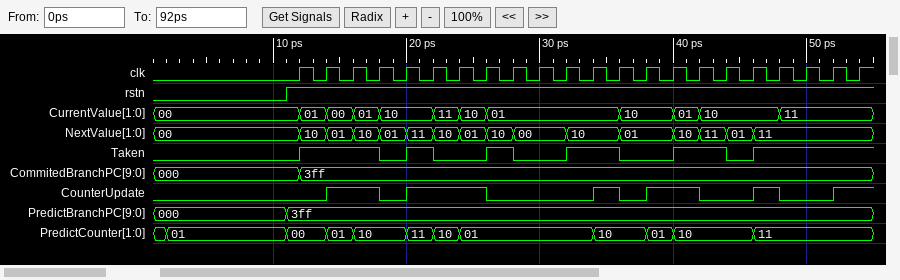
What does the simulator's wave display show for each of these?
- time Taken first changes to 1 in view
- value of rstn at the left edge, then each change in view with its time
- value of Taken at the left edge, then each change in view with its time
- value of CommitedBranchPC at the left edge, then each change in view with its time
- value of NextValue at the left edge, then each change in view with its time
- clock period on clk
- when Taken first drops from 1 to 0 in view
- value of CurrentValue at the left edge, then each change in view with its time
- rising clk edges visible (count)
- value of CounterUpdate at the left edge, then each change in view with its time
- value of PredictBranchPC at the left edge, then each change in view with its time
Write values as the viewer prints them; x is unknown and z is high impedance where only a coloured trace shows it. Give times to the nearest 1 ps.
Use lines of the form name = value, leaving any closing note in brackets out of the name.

time Taken first changes to 1 in view = 12 ps
value of rstn at the left edge, then each change in view with its time = 0, 1 at 11 ps
value of Taken at the left edge, then each change in view with its time = 0, 1 at 12 ps, 0 at 18 ps, 1 at 20 ps, 0 at 22 ps, 1 at 26 ps, 0 at 28 ps, 1 at 32 ps, 0 at 36 ps, 1 at 40 ps, 0 at 44 ps, 1 at 46 ps
value of CommitedBranchPC at the left edge, then each change in view with its time = 000, 3ff at 12 ps
value of NextValue at the left edge, then each change in view with its time = 00, 10 at 12 ps, 01 at 14 ps, 10 at 16 ps, 01 at 18 ps, 11 at 20 ps, 10 at 22 ps, 01 at 24 ps, 10 at 26 ps, 00 at 28 ps, 10 at 32 ps, 01 at 36 ps, 10 at 40 ps, 11 at 42 ps, 01 at 44 ps, 11 at 46 ps
clock period on clk = 2 ps
when Taken first drops from 1 to 0 in view = 18 ps
value of CurrentValue at the left edge, then each change in view with its time = 00, 01 at 12 ps, 00 at 14 ps, 01 at 16 ps, 10 at 18 ps, 11 at 22 ps, 10 at 24 ps, 01 at 26 ps, 10 at 36 ps, 01 at 40 ps, 10 at 42 ps, 11 at 48 ps
rising clk edges visible = 22
value of CounterUpdate at the left edge, then each change in view with its time = 0, 1 at 14 ps, 0 at 18 ps, 1 at 20 ps, 0 at 26 ps, 1 at 34 ps, 0 at 36 ps, 1 at 38 ps, 0 at 42 ps, 1 at 46 ps, 0 at 48 ps, 1 at 52 ps
value of PredictBranchPC at the left edge, then each change in view with its time = 000, 3ff at 11 ps
